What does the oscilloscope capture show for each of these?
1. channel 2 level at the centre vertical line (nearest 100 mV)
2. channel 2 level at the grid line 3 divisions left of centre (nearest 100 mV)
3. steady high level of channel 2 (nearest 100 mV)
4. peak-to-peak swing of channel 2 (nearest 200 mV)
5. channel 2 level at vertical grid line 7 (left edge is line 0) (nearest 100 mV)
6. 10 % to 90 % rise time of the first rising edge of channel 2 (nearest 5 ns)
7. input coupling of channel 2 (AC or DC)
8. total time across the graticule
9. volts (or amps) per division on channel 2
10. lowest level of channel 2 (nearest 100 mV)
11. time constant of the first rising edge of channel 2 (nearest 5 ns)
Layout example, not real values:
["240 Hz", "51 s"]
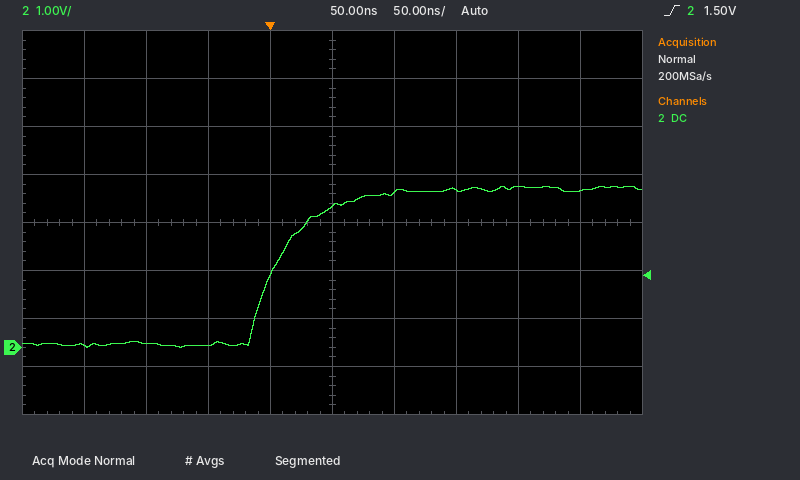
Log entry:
["2.9 V", "100 mV", "3.3 V", "3.4 V", "3.3 V", "65 ns", "DC", "500 ns", "1 V", "0.0 V", "30 ns"]
